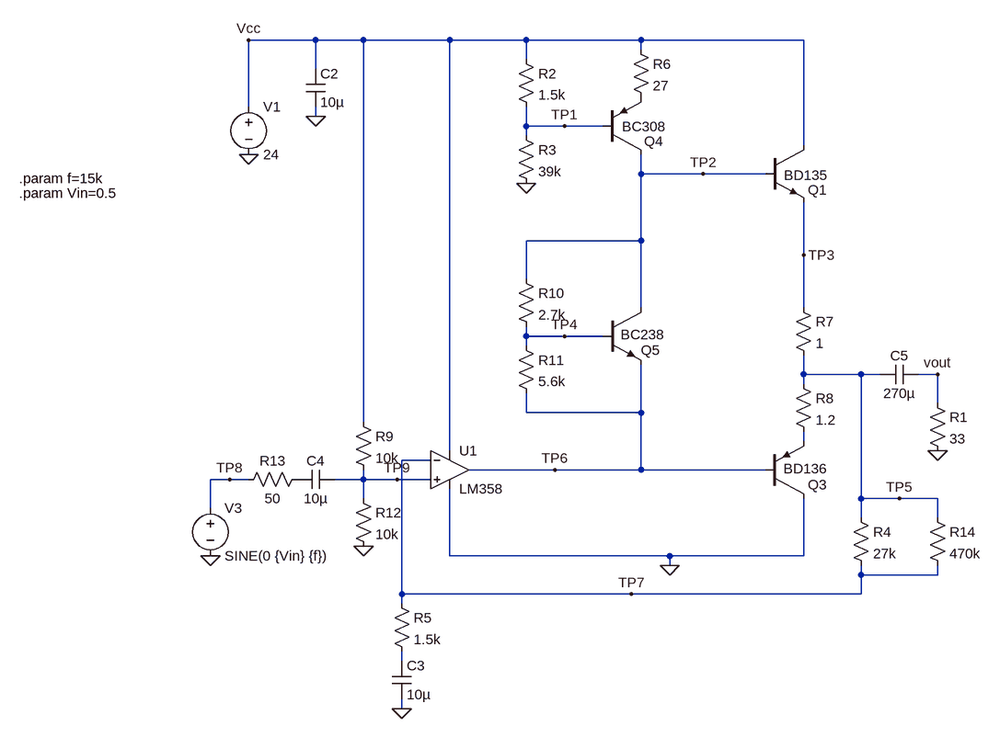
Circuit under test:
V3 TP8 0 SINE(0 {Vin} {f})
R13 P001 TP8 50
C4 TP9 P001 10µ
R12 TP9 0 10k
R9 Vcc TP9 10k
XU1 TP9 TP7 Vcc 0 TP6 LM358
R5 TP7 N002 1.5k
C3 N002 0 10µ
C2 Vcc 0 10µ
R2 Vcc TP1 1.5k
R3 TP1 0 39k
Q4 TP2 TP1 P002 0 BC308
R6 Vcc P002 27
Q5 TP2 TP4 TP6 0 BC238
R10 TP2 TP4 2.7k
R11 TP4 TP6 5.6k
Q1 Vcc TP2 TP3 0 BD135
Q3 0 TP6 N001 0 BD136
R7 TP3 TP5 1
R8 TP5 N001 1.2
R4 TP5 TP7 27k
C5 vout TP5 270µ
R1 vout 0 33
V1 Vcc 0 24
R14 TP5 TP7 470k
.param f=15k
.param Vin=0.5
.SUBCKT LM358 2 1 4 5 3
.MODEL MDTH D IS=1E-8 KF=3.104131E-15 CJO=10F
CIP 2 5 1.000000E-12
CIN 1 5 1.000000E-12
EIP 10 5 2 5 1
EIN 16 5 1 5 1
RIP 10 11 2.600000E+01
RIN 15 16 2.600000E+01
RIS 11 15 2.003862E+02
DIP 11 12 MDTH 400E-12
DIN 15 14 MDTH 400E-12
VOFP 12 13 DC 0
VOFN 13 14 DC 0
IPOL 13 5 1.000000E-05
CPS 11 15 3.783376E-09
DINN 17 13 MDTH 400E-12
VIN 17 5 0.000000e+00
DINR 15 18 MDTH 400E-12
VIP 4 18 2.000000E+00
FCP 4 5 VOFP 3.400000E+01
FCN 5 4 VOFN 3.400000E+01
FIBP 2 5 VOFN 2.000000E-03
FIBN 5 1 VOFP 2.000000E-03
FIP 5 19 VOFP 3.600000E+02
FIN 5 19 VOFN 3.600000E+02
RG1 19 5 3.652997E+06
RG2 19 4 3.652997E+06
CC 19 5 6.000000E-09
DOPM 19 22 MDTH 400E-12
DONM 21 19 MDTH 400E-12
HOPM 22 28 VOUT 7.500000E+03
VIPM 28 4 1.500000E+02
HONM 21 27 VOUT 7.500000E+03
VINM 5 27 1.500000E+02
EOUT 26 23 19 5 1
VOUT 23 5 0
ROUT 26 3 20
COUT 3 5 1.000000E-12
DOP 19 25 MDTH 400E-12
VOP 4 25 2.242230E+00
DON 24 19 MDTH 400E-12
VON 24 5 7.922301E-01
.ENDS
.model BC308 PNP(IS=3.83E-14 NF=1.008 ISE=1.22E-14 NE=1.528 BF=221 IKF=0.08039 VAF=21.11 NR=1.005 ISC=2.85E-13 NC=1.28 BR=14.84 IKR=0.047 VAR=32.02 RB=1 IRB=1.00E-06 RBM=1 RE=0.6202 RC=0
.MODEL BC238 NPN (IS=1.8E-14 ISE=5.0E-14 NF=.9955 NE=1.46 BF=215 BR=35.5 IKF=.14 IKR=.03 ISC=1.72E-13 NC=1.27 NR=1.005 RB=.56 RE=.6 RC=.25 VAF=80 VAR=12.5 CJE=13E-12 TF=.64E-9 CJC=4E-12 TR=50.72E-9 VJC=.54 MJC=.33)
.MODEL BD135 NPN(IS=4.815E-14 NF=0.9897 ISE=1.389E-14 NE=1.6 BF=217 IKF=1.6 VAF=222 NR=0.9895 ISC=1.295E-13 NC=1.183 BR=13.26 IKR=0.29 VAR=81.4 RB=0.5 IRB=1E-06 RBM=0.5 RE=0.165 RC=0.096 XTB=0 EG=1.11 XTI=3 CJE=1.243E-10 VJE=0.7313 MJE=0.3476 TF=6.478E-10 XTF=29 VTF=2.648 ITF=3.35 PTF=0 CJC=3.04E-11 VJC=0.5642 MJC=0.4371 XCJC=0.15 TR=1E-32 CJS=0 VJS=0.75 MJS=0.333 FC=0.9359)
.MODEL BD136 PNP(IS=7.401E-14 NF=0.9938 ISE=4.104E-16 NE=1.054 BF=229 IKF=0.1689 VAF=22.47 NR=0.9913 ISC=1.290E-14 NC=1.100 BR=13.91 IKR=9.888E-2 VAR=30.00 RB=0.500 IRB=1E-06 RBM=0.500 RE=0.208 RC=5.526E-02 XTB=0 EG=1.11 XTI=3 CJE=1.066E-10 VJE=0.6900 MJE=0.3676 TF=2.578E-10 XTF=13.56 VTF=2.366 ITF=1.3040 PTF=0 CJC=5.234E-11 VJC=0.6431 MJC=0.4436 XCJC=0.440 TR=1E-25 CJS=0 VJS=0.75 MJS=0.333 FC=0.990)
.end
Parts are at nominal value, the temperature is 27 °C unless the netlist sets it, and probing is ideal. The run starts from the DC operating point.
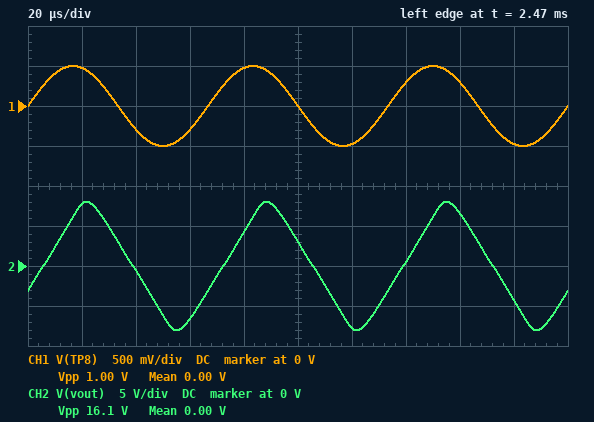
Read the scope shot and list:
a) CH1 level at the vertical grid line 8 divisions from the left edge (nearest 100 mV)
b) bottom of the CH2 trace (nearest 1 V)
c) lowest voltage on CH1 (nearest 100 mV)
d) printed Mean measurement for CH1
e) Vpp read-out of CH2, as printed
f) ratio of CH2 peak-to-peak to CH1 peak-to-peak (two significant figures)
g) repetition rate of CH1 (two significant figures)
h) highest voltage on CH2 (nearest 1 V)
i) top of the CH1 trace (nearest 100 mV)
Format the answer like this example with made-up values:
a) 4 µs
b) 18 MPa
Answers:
a) 300 mV
b) -8 V
c) -500 mV
d) 0.00 V
e) 16.1 V
f) 16
g) 15 kHz
h) 8 V
i) 500 mV
